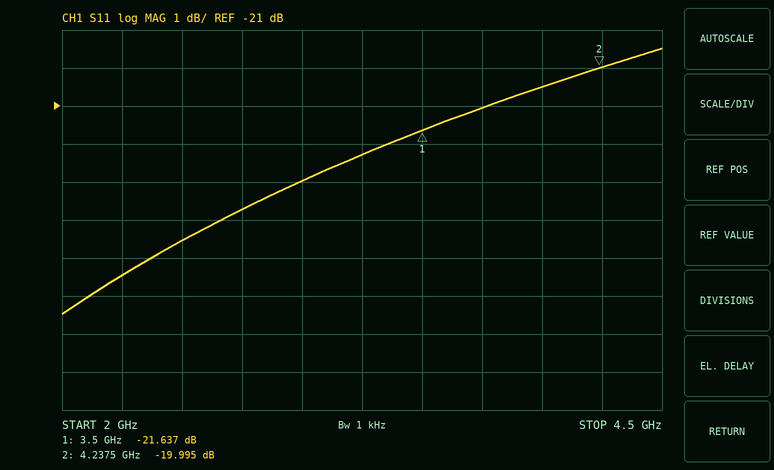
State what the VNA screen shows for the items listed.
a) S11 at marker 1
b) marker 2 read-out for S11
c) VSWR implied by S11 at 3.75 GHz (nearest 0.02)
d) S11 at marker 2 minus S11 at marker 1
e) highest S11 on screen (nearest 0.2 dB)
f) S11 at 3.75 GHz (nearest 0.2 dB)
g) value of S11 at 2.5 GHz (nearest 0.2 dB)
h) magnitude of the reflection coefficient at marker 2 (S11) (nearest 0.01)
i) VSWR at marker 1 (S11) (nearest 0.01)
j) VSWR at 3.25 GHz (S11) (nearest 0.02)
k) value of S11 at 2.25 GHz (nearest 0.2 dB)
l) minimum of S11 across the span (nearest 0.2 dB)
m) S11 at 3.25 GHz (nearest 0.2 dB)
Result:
-21.637 dB
-19.995 dB
1.20
1.642 dB
-19.4 dB
-21.0 dB
-24.6 dB
0.10
1.18
1.16
-25.4 dB
-26.4 dB
-22.2 dB
